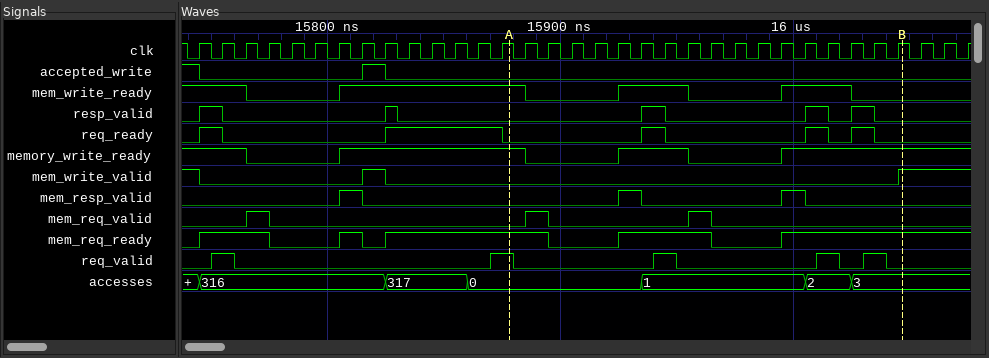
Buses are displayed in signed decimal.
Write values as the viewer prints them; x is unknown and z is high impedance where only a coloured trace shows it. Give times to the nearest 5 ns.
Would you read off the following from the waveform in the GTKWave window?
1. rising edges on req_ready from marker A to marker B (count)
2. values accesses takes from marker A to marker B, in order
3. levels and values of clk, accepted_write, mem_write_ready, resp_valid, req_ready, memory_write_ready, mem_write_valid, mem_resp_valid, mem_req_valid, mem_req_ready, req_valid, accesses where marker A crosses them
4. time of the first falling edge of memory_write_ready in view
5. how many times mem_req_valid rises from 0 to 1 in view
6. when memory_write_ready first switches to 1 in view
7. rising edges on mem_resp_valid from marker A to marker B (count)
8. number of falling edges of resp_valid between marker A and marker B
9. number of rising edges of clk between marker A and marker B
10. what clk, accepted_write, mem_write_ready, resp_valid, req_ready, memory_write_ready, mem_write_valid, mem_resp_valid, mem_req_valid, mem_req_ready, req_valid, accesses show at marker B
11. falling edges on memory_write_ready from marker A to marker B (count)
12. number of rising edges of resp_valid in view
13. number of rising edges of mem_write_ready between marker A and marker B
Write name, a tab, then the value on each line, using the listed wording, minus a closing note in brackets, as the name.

rising edges on req_ready from marker A to marker B	3
values accesses takes from marker A to marker B, in order	0, 1, 2, 3
levels and values of clk, accepted_write, mem_write_ready, resp_valid, req_ready, memory_write_ready, mem_write_valid, mem_resp_valid, mem_req_valid, mem_req_ready, req_valid, accesses where marker A crosses them	clk=1, accepted_write=0, mem_write_ready=1, resp_valid=0, req_ready=0, memory_write_ready=1, mem_write_valid=0, mem_resp_valid=0, mem_req_valid=0, mem_req_ready=1, req_valid=1, accesses=0
time of the first falling edge of memory_write_ready in view	15765 ns
how many times mem_req_valid rises from 0 to 1 in view	3
when memory_write_ready first switches to 1 in view	15805 ns
rising edges on mem_resp_valid from marker A to marker B	2
number of falling edges of resp_valid between marker A and marker B	3
number of rising edges of clk between marker A and marker B	17
what clk, accepted_write, mem_write_ready, resp_valid, req_ready, memory_write_ready, mem_write_valid, mem_resp_valid, mem_req_valid, mem_req_ready, req_valid, accesses show at marker B	clk=1, accepted_write=0, mem_write_ready=0, resp_valid=0, req_ready=0, memory_write_ready=1, mem_write_valid=1, mem_resp_valid=0, mem_req_valid=0, mem_req_ready=1, req_valid=0, accesses=3
falling edges on memory_write_ready from marker A to marker B	2
number of rising edges of resp_valid in view	5
number of rising edges of mem_write_ready between marker A and marker B	2
